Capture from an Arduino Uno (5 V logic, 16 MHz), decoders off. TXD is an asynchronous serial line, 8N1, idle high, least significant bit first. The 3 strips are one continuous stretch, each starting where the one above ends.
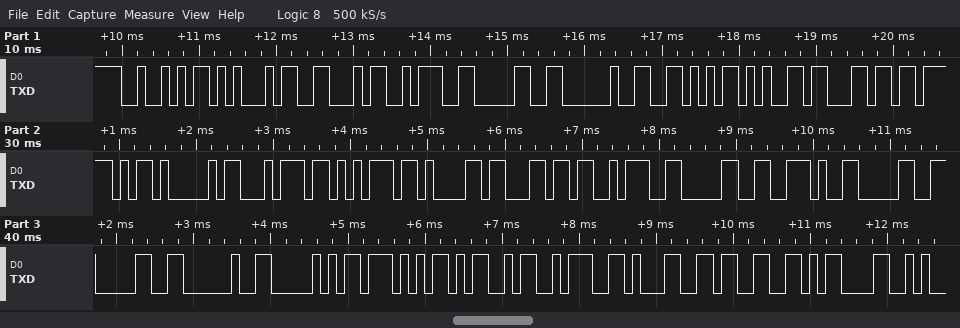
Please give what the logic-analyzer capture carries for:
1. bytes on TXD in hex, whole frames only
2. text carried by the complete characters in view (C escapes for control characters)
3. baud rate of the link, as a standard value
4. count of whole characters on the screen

52 45 46 3A 30 20 56 65 6C 5F 41 74 75 61 6C 3A 30 2E 30 30 20 50 57 4D 3A 31 33 0D
"REF:0 Vel_Atual:0.00 PWM:13\r"
9600 baud
28
